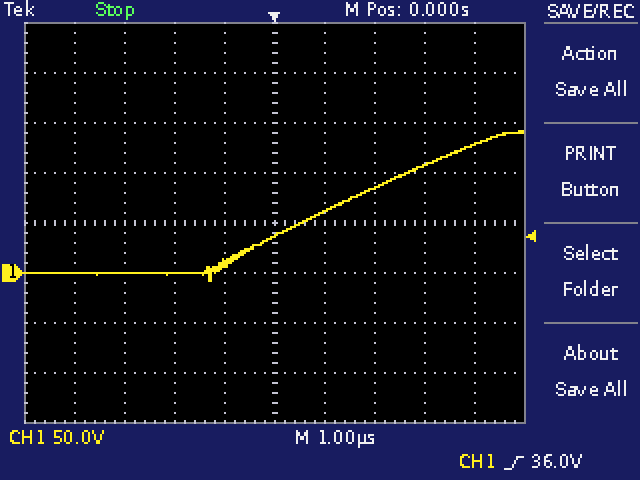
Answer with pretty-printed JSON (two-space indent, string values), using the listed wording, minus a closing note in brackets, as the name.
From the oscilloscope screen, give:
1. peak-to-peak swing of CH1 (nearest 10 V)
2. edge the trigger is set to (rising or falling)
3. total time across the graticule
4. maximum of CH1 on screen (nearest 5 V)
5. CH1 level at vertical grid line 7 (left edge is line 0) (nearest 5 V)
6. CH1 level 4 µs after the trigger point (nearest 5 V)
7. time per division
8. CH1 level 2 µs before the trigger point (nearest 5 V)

{
  "peak-to-peak swing of CH1": "150 V",
  "edge the trigger is set to": "rising",
  "total time across the graticule": "10 µs",
  "maximum of CH1 on screen": "140 V",
  "CH1 level at vertical grid line 7 (left edge is line 0)": "85 V",
  "CH1 level 4 µs after the trigger point": "130 V",
  "time per division": "1 µs",
  "CH1 level 2 µs before the trigger point": "0 V"
}
